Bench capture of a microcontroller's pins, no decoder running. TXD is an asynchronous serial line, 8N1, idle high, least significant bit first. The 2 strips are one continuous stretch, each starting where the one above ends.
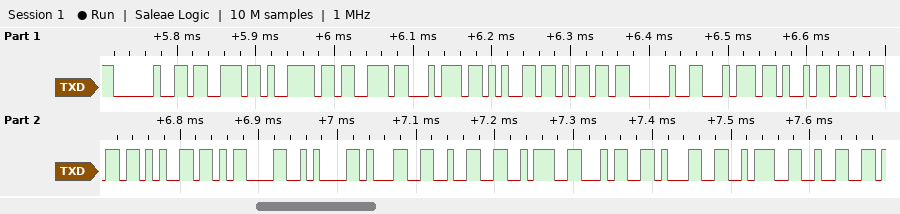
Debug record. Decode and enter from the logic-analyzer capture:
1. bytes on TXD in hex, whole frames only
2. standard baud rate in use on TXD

20 73 79 73 74 65 6D 20 74 69 6D 65 0D 0A 31 32 3A 34 31 3A 32
115200 baud
